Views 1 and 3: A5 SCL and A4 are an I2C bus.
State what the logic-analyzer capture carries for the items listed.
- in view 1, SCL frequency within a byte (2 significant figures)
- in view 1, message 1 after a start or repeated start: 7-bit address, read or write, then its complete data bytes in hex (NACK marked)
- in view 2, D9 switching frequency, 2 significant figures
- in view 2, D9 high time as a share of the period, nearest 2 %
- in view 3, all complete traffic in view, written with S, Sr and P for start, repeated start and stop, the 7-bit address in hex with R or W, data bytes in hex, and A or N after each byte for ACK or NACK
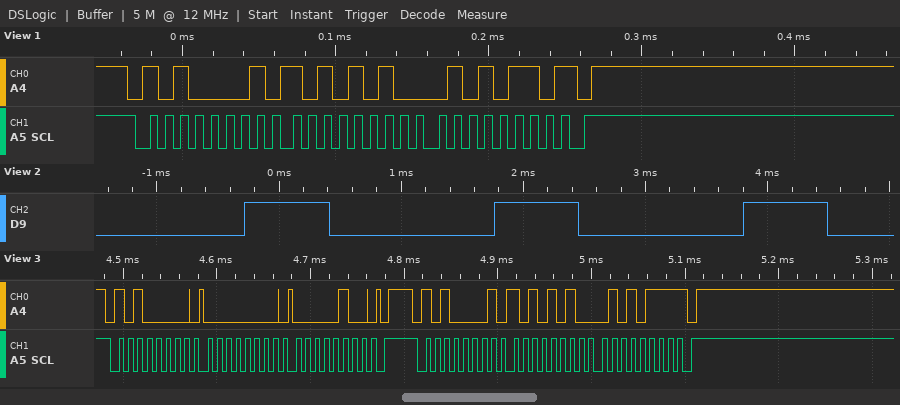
100 kHz
0x50 read: AA 56 NACK
490 Hz
34 %
S 50W A 00 A 04 A P S 50R A AA A 57 N P
